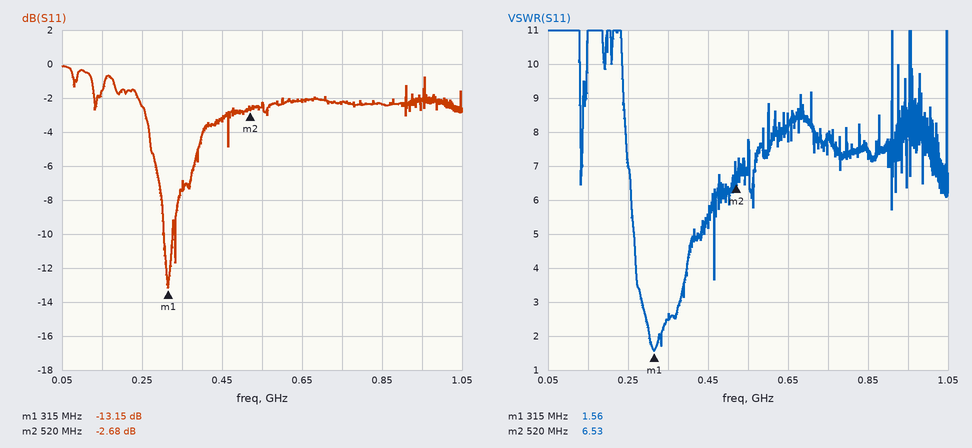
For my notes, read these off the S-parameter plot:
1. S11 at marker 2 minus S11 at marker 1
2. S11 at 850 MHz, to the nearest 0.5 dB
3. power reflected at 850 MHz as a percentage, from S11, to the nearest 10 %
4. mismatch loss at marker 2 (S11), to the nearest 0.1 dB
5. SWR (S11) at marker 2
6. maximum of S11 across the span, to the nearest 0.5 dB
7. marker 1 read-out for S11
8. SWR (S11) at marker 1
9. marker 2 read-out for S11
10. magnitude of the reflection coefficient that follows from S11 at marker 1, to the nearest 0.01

10.47 dB
-2.5 dB
60 %
3.4 dB
6.53
0.0 dB
-13.15 dB
1.56
-2.68 dB
0.22
